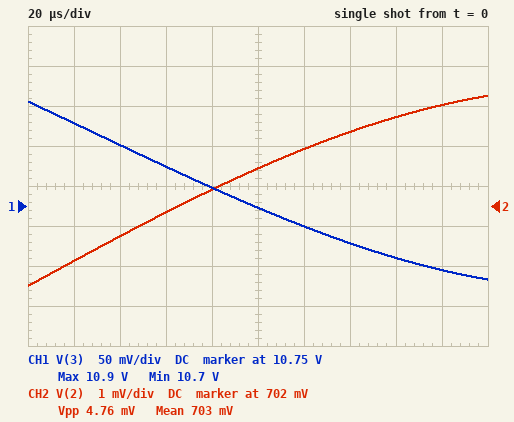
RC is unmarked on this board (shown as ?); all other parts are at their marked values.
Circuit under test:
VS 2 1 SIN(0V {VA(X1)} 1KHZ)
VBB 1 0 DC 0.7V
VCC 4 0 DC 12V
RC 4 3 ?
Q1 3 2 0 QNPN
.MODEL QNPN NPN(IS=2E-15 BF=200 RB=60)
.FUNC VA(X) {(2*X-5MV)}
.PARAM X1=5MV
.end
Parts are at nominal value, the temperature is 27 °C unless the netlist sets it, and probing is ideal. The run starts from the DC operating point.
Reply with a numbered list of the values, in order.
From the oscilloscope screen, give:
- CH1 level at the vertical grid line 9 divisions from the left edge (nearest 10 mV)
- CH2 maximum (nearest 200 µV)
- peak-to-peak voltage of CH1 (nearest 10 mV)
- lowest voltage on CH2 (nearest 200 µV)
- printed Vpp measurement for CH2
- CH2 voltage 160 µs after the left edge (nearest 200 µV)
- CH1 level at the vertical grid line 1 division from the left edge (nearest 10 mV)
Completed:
1. 10.67 V
2. 704.8 mV
3. 220 mV
4. 700.0 mV
5. 4.76 mV
6. 704.2 mV
7. 10.85 V
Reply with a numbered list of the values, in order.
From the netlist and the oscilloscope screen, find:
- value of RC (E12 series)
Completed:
1. 1 kΩ
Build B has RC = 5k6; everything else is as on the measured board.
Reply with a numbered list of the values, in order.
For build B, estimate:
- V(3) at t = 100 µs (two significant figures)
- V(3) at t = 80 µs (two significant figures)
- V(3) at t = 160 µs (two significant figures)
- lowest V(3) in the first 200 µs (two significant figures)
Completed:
1. 5.0 V
2. 5.1 V
3. 4.6 V
4. 4.5 V
